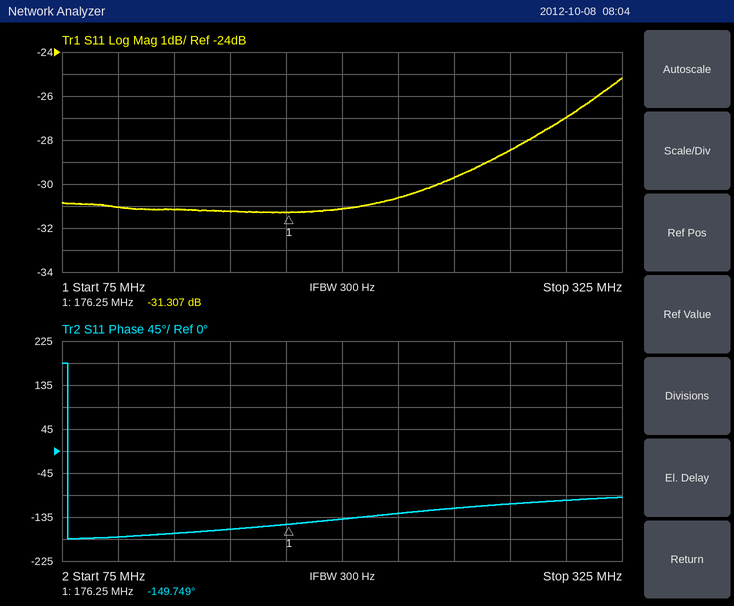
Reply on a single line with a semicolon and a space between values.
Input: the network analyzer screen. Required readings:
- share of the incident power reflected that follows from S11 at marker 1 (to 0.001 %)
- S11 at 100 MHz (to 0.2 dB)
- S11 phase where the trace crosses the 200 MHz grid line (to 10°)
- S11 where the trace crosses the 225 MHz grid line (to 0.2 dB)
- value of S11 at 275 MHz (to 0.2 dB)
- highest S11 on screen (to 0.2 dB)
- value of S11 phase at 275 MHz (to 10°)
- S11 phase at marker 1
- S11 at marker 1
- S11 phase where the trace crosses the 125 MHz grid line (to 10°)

0.074 %; -31.0 dB; -140°; -30.6 dB; -28.4 dB; -25.2 dB; -110°; -149.749°; -31.307 dB; -170°
